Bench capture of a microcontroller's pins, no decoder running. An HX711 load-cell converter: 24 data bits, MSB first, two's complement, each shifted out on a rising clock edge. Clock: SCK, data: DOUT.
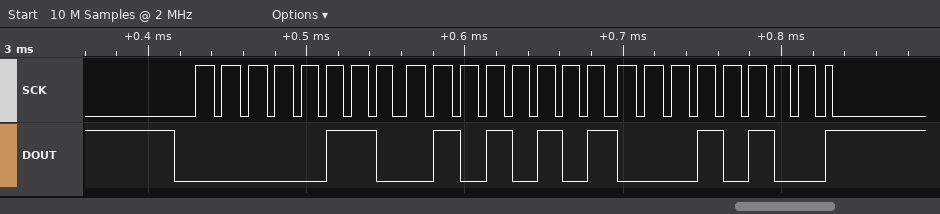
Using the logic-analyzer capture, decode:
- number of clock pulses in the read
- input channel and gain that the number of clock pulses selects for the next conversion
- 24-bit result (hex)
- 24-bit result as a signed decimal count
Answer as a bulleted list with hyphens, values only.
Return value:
- 25
- channel A, gain 128
- 0x065514
- 414996
